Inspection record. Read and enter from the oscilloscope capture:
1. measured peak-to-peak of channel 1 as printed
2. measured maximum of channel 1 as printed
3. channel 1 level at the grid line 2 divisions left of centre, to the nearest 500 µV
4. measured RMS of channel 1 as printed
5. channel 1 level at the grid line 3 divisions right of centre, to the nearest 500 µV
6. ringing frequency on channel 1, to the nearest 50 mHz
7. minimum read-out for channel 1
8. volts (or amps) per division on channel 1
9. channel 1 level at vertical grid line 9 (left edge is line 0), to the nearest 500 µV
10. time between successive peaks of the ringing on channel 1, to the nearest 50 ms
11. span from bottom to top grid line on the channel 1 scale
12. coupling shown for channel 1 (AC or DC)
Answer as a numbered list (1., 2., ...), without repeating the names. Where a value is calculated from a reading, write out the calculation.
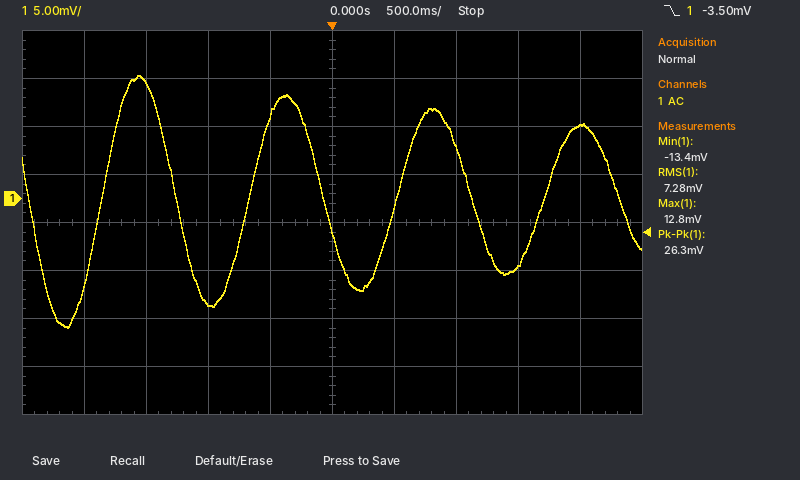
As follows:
1. 26.3 mV
2. 12.8 mV
3. -11.0 mV
4. 7.28 mV
5. -7.0 mV
6. 1 / 1.20 s ≈ 833 mHz, so 850 mHz to the nearest 50 mHz
7. -13.4 mV
8. 5 mV
9. 7.5 mV
10. 1.20 s
11. 40 mV
12. AC
